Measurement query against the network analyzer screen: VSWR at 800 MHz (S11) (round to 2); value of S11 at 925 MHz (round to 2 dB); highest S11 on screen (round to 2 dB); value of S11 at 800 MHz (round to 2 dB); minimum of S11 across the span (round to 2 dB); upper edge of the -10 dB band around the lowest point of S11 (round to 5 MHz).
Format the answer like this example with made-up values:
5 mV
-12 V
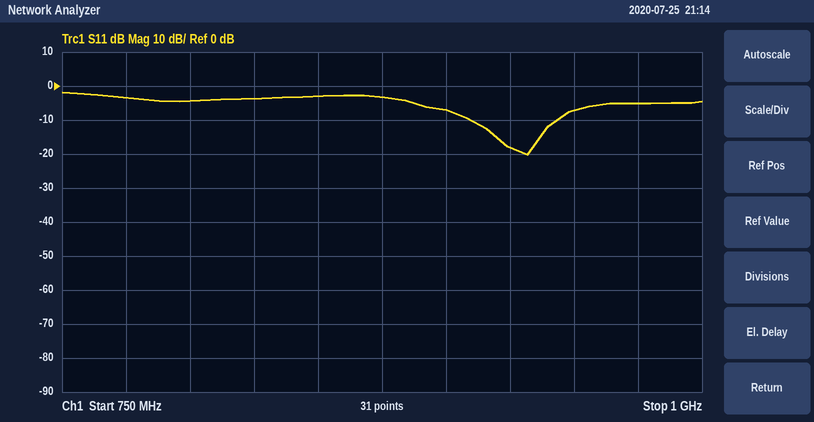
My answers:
4
-18 dB
-2 dB
-4 dB
-20 dB
945 MHz
